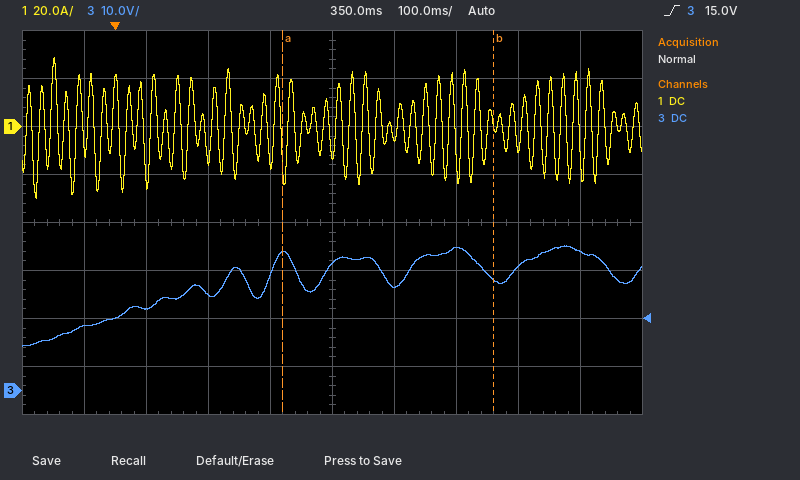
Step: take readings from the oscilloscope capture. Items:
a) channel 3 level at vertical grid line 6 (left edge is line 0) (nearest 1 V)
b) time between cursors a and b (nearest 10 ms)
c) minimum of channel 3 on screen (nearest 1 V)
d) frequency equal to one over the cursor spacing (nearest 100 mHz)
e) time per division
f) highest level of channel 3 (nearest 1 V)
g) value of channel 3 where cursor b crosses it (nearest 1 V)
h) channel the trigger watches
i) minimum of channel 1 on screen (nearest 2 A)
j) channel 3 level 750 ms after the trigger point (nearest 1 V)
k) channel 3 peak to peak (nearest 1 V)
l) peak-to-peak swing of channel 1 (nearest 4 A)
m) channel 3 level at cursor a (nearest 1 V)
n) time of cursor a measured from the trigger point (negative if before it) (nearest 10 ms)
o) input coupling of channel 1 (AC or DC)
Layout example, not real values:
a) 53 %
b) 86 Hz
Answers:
a) 22 V
b) 340 ms
c) 9 V
d) 2.9 Hz
e) 100 ms
f) 30 V
g) 23 V
h) channel 3
i) -30 A
j) 29 V
k) 21 V
l) 60 A
m) 29 V
n) +270 ms
o) DC
